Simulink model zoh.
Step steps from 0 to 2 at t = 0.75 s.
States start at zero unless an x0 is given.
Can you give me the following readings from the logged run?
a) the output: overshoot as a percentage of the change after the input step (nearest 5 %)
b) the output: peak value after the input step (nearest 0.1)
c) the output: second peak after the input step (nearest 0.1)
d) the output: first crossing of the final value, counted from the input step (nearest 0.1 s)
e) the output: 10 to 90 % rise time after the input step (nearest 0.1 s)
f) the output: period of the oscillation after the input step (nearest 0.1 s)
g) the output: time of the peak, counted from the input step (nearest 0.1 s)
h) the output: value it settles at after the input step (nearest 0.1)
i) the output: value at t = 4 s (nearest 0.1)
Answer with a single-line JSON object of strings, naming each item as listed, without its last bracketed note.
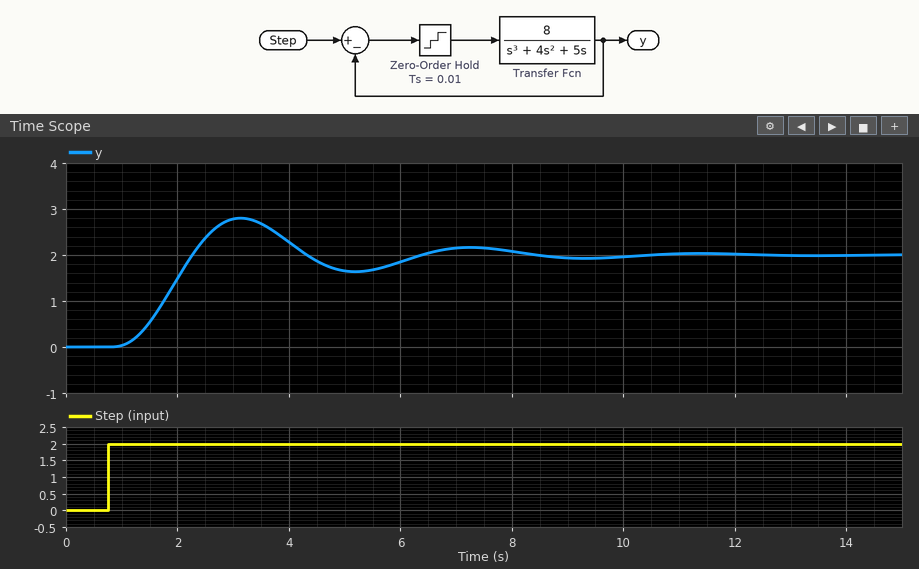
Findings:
{"the output: overshoot as a percentage of the change after the input step": "40 %", "the output: peak value after the input step": "2.8", "the output: second peak after the input step": "2.2", "the output: first crossing of the final value, counted from the input step": "1.5 s", "the output: 10 to 90 % rise time after the input step": "0.9 s", "the output: period of the oscillation after the input step": "4.1 s", "the output: time of the peak, counted from the input step": "2.4 s", "the output: value it settles at after the input step": "2.0", "the output: value at t = 4 s": "2.3"}
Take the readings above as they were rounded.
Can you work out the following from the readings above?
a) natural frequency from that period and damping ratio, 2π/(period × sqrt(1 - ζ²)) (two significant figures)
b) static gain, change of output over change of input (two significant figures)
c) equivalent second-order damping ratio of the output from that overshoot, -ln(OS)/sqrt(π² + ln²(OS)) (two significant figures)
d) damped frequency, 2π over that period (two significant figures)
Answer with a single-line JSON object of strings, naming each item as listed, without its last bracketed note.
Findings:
{"natural frequency from that period and damping ratio, 2π/(period × sqrt(1 - ζ²))": "1.6 rad/s", "static gain, change of output over change of input": "1.0", "equivalent second-order damping ratio of the output from that overshoot, -ln(OS)/sqrt(π² + ln²(OS))": "0.28", "damped frequency, 2π over that period": "1.5 rad/s"}
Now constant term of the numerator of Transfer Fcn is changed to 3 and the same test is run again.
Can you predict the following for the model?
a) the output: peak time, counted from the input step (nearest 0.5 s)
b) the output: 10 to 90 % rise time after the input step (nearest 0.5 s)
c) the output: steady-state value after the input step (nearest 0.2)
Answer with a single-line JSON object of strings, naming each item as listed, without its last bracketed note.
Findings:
{"the output: peak time, counted from the input step": "4.5 s", "the output: 10 to 90 % rise time after the input step": "2.0 s", "the output: steady-state value after the input step": "2.0"}
